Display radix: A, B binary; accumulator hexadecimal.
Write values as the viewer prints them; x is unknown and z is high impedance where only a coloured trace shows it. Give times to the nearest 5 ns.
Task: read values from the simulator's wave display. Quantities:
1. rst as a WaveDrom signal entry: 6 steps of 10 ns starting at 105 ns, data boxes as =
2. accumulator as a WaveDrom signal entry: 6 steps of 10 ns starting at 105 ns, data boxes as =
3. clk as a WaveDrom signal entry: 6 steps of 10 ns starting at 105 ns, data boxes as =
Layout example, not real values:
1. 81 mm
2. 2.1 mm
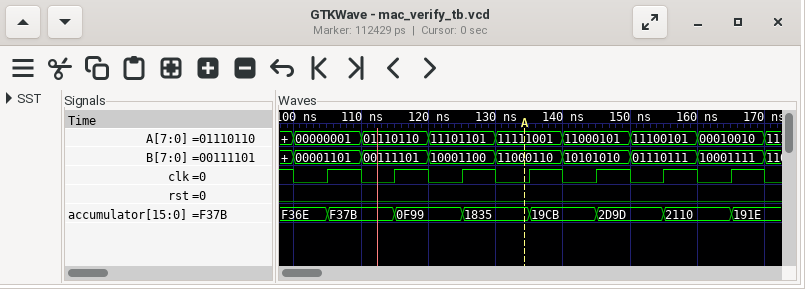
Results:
1. {name: 'rst', wave: '0.....'}
2. {name: 'accumulator', wave: '======', data: 'F37B 0F99 1835 19CB 2D9D 2110'}
3. {name: 'clk', wave: 'p.....'}
